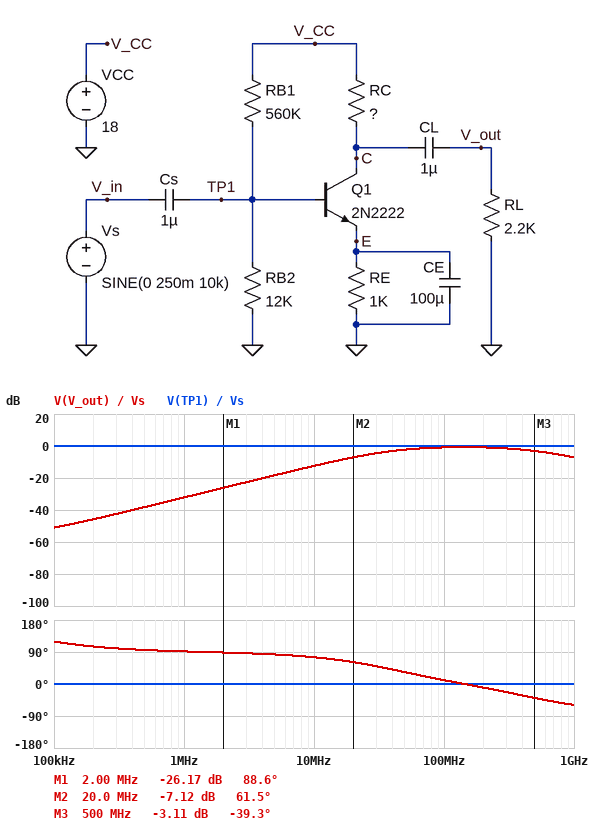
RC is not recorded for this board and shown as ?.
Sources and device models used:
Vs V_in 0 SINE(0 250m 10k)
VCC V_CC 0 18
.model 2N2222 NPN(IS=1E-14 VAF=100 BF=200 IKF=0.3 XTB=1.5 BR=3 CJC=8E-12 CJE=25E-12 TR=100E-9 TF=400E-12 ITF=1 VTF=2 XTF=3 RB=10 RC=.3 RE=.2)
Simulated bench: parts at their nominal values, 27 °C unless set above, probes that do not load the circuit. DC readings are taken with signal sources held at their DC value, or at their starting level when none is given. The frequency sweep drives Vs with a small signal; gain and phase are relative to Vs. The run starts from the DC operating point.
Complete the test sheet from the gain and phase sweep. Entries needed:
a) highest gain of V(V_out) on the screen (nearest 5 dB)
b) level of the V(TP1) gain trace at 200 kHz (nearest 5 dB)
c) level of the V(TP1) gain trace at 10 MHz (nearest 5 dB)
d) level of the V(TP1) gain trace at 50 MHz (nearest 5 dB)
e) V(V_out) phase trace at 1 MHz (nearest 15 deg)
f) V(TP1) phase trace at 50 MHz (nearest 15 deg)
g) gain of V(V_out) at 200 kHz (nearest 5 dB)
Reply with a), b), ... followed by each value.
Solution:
a) 0 dB
b) 0 dB
c) 0 dB
d) 0 dB
e) 90 deg
f) 0 deg
g) -45 dB
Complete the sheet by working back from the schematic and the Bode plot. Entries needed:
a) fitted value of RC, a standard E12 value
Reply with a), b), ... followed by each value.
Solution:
a) 3.9 kΩ
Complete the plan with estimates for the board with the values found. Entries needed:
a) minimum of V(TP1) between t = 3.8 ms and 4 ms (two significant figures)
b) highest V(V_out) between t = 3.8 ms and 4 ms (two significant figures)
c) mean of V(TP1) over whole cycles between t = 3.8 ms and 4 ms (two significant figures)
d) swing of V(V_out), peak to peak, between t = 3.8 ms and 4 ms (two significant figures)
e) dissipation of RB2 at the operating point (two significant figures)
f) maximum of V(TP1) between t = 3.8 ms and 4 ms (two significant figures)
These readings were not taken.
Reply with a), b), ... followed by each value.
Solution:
a) 130 mV
b) 33 mV
c) 380 mV
d) 510 mV
e) 12 µW
f) 630 mV
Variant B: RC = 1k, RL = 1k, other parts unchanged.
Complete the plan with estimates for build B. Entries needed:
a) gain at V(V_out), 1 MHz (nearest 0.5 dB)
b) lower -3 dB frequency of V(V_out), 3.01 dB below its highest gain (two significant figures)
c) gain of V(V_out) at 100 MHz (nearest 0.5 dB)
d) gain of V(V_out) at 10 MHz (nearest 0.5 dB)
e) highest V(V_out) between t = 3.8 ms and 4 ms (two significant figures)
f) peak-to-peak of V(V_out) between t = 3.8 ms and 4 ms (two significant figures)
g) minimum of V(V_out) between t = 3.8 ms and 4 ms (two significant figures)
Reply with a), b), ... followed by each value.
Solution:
a) -41.0 dB
b) 81 MHz
c) -4.0 dB
d) -21.0 dB
e) 21 mV
f) 180 mV
g) -160 mV
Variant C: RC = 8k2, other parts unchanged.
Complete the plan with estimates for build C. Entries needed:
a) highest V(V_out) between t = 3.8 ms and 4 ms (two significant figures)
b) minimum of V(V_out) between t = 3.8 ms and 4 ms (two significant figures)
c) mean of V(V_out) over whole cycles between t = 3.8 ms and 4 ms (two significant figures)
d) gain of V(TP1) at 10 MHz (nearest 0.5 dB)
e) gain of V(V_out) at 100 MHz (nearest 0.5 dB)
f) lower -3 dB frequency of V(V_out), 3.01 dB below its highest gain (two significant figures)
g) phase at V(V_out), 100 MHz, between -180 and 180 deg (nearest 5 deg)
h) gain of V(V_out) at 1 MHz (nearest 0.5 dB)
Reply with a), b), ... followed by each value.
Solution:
a) 27 mV
b) -600 mV
c) -55 mV
d) 0 dB
e) -0.5 dB
f) 29 MHz
g) 5 deg
h) -30.5 dB
